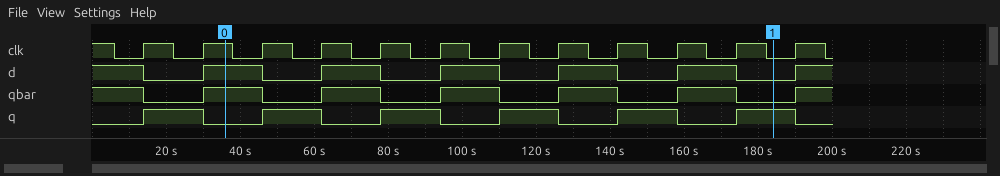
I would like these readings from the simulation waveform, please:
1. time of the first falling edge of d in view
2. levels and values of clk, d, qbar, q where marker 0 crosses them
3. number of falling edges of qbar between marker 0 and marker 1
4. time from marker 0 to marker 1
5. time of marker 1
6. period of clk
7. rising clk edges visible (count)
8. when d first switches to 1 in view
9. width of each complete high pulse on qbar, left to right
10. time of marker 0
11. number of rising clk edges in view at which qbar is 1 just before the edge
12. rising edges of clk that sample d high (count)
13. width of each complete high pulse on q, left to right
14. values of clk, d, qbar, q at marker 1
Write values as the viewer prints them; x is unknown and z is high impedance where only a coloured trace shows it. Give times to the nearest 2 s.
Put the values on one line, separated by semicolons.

14 s; clk=1, d=1, qbar=1, q=0; 5; 148 s; 184 s; 16 s; 12; 30 s; 16 s, 16 s, 16 s, 16 s, 16 s; 36 s; 6; 6; 16 s, 16 s, 16 s, 16 s, 16 s, 16 s; clk=0, d=0, qbar=0, q=1
